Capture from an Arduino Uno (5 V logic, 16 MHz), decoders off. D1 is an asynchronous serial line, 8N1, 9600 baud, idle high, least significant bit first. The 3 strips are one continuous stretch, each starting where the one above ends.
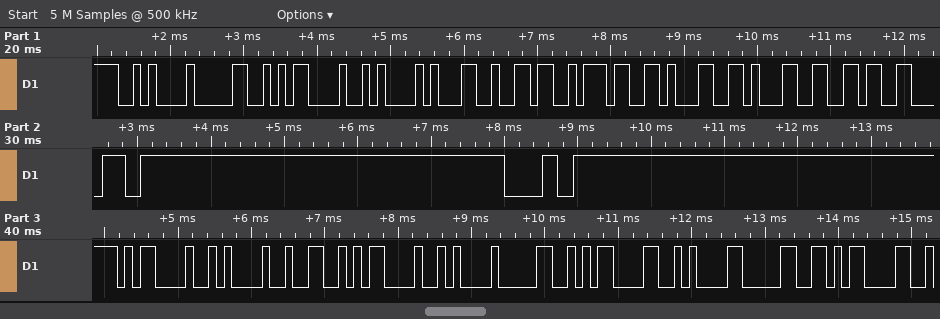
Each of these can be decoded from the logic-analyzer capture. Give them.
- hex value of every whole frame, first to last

0x0A 0x30 0x0D 0x0A 0x31 0x36 0x37 0x31 0x31 0x36 0x38 0x30 0x0D 0x0A 0x32 0x0D 0x0A 0x30 0x0D 0x0A 0x30 0x0D
